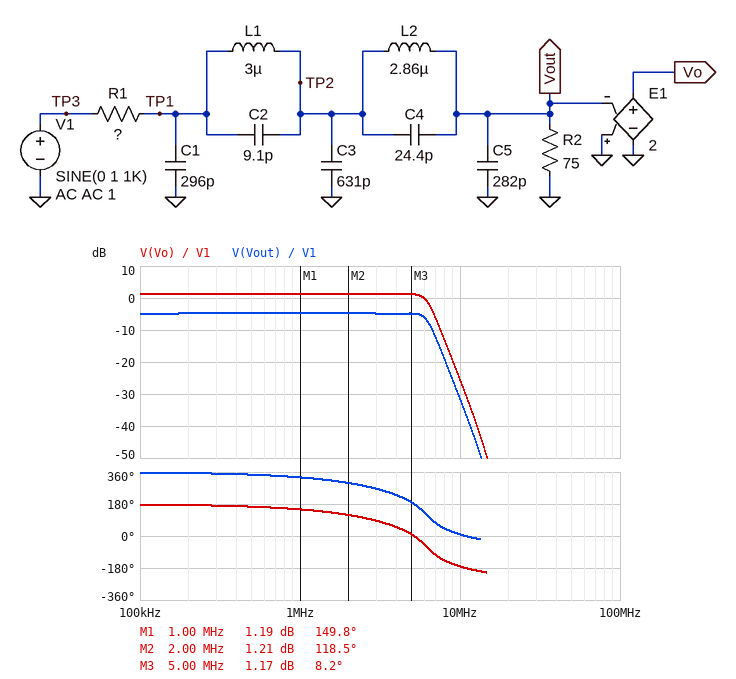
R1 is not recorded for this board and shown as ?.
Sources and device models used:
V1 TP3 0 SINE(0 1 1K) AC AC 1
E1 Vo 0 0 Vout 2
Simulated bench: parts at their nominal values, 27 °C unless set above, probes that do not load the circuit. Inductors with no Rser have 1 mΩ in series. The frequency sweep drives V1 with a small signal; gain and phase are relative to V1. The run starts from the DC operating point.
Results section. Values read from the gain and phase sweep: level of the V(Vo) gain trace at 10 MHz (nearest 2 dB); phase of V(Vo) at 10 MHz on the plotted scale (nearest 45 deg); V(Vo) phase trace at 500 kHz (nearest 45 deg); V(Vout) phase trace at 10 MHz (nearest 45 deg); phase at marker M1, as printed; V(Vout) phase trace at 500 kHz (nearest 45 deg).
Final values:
-26 dB
-180 deg
180 deg
0 deg
149.8 deg
360 deg
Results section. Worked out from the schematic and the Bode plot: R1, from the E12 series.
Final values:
56 Ω
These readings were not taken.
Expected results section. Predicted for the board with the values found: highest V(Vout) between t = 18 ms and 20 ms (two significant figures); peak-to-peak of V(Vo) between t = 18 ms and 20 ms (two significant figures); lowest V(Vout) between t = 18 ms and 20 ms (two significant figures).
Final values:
570 mV
2.3 V
-570 mV
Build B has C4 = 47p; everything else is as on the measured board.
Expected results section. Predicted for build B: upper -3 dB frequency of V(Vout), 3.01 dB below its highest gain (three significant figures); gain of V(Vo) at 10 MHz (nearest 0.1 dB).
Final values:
6.17 MHz
-30.2 dB
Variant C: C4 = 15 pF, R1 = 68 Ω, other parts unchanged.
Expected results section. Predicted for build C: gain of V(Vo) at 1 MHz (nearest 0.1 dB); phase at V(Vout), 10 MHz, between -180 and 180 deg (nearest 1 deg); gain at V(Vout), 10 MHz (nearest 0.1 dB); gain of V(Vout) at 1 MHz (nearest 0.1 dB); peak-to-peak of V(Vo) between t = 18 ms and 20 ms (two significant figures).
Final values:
0.4 dB
5 deg
-30.6 dB
-5.6 dB
2.1 V
